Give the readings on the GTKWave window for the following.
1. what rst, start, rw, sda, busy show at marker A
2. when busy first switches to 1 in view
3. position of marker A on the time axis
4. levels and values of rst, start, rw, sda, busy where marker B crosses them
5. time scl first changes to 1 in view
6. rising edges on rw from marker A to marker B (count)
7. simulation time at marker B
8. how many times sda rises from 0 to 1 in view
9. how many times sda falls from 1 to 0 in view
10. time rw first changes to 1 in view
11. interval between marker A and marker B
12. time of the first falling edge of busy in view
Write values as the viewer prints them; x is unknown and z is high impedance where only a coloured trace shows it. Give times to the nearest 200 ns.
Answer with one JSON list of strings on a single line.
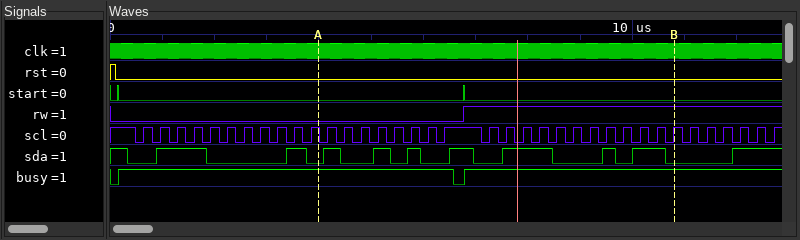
["rst=0, start=0, rw=0, sda=0, busy=1", "200 ns", "4000 ns", "rst=0, start=0, rw=1, sda=0, busy=1", "600 ns", "1", "10800 ns", "10", "10", "6800 ns", "6800 ns", "6600 ns"]
